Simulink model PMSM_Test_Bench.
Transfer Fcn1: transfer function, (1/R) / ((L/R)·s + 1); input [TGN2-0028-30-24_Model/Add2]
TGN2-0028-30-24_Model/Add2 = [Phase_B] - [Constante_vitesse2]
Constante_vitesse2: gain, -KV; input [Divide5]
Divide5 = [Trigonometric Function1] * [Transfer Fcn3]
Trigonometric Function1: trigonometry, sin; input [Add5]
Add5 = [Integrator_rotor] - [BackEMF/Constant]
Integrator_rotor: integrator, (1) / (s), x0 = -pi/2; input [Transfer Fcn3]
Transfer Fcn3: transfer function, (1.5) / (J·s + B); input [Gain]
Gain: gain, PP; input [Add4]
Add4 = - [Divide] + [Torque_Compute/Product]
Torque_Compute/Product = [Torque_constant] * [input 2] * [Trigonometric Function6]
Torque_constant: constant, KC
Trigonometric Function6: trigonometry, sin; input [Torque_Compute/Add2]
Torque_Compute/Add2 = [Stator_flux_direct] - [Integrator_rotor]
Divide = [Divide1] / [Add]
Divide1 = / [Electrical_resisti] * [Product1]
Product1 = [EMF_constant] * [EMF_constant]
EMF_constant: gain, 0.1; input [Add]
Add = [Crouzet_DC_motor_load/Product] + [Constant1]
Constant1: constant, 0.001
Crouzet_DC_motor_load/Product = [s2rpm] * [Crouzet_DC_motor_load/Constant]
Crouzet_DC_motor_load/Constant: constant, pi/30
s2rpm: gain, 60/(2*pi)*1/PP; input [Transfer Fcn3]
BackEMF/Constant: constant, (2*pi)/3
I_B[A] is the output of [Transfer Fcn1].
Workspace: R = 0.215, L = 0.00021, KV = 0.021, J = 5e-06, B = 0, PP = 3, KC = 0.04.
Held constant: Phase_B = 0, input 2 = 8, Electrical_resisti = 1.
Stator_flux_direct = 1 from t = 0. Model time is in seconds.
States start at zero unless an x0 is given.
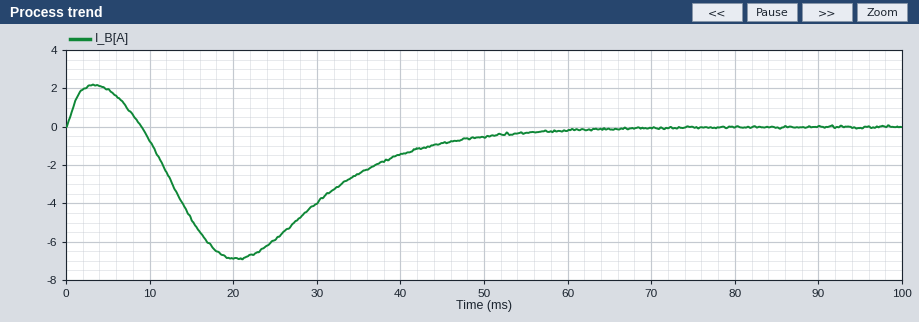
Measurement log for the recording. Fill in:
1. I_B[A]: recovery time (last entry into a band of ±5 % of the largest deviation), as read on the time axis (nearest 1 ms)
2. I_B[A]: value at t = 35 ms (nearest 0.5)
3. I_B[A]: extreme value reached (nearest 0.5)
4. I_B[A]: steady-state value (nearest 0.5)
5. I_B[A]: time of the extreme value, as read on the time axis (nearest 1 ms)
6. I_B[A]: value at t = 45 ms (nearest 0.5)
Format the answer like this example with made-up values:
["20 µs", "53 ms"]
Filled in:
["54 ms", "-2.5", "-7.0", "0.0", "20 ms", "-1.0"]
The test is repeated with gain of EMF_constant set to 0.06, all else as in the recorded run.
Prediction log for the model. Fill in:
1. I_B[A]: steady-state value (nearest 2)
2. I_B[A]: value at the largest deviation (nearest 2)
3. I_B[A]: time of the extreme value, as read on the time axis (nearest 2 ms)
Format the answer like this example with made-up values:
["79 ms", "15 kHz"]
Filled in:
["0", "-20", "10 ms"]
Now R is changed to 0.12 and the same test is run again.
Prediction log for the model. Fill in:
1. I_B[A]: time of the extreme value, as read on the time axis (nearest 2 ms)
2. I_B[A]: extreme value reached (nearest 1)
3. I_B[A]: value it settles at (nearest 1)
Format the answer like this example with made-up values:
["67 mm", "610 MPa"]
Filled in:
["22 ms", "-12", "0"]
